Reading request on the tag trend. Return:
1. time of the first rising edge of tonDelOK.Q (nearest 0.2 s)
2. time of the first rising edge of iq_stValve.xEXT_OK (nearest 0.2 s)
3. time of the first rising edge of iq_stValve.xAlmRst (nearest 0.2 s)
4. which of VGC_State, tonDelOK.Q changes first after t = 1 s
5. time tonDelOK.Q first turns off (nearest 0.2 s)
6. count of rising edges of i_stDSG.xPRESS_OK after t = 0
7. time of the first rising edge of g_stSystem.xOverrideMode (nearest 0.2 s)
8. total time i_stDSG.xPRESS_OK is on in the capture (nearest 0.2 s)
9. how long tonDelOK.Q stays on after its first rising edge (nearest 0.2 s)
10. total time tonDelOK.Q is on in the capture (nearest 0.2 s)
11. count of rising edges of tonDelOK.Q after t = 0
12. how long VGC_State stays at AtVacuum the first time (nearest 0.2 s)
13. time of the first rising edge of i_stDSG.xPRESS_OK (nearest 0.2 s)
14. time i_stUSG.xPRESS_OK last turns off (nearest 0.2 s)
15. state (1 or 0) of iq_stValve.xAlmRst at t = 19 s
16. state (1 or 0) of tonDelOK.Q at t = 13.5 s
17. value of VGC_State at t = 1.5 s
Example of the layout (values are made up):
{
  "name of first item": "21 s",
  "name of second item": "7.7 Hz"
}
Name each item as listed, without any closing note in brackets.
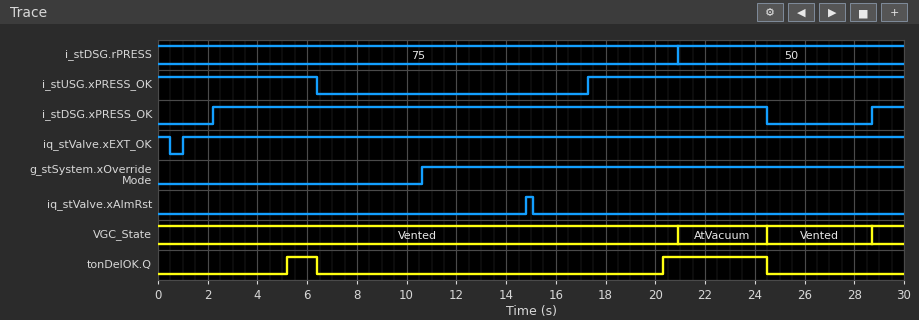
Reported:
{
  "time of the first rising edge of tonDelOK.Q": "5.2 s",
  "time of the first rising edge of iq_stValve.xEXT_OK": "1.0 s",
  "time of the first rising edge of iq_stValve.xAlmRst": "14.8 s",
  "which of VGC_State, tonDelOK.Q changes first after t = 1 s": "tonDelOK.Q",
  "time tonDelOK.Q first turns off": "6.4 s",
  "count of rising edges of i_stDSG.xPRESS_OK after t = 0": "2",
  "time of the first rising edge of g_stSystem.xOverrideMode": "10.6 s",
  "total time i_stDSG.xPRESS_OK is on in the capture": "23.6 s",
  "how long tonDelOK.Q stays on after its first rising edge": "1.2 s",
  "total time tonDelOK.Q is on in the capture": "5.4 s",
  "count of rising edges of tonDelOK.Q after t = 0": "2",
  "how long VGC_State stays at AtVacuum the first time": "3.6 s",
  "time of the first rising edge of i_stDSG.xPRESS_OK": "2.2 s",
  "time i_stUSG.xPRESS_OK last turns off": "6.4 s",
  "state (1 or 0) of iq_stValve.xAlmRst at t = 19 s": "0",
  "state (1 or 0) of tonDelOK.Q at t = 13.5 s": "0",
  "value of VGC_State at t = 1.5 s": "Vented"
}
